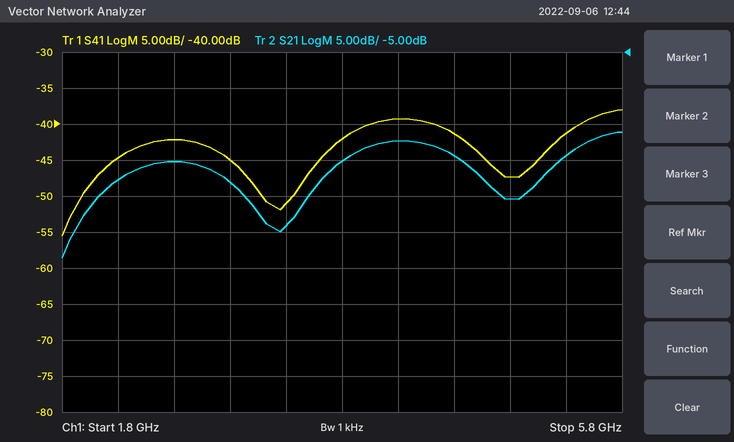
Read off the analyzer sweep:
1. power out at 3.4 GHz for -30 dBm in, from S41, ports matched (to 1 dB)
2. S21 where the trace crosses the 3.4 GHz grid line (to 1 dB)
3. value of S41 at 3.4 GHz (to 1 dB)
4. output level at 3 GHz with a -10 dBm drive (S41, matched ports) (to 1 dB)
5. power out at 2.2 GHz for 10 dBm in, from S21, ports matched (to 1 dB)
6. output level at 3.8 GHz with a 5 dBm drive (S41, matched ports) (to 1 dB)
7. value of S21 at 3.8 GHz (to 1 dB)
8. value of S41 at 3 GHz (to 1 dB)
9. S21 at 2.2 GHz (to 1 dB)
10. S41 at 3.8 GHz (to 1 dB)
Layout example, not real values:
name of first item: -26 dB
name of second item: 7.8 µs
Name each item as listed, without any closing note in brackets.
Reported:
power out at 3.4 GHz for -30 dBm in, from S41, ports matched: -81 dBm
S21 where the trace crosses the 3.4 GHz grid line: -29 dB
value of S41 at 3.4 GHz: -51 dB
output level at 3 GHz with a -10 dBm drive (S41, matched ports): -55 dBm
power out at 2.2 GHz for 10 dBm in, from S21, ports matched: -13 dBm
output level at 3.8 GHz with a 5 dBm drive (S41, matched ports): -37 dBm
value of S21 at 3.8 GHz: -20 dB
value of S41 at 3 GHz: -45 dB
S21 at 2.2 GHz: -23 dB
S41 at 3.8 GHz: -42 dB
